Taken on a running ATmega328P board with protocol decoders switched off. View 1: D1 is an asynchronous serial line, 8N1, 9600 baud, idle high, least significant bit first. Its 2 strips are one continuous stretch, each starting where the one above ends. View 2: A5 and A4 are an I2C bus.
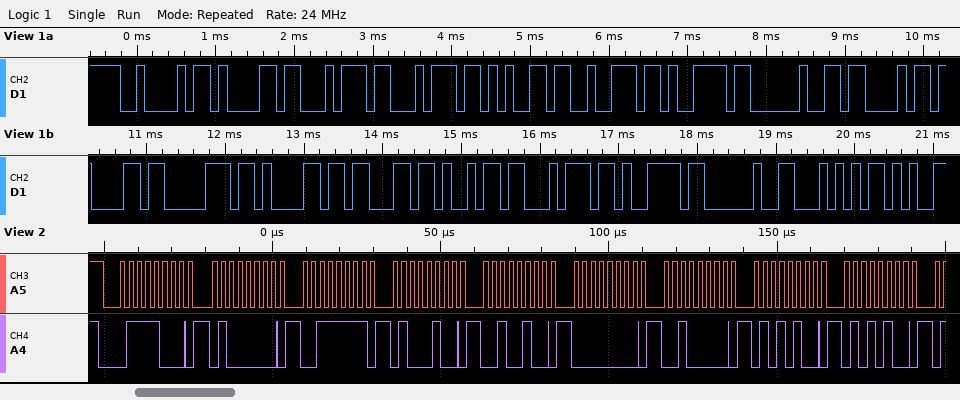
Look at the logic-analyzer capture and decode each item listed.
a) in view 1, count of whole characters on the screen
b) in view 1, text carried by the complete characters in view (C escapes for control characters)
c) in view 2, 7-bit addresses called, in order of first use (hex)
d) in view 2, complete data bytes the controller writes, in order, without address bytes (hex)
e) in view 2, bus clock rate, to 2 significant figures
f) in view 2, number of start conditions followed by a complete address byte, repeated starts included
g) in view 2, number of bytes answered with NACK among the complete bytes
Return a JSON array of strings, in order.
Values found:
["18", "\"Battery Capacity T\"", "0x3C", "40 3F 44 24 00 20 54 54", "400 kHz", "1", "0"]
